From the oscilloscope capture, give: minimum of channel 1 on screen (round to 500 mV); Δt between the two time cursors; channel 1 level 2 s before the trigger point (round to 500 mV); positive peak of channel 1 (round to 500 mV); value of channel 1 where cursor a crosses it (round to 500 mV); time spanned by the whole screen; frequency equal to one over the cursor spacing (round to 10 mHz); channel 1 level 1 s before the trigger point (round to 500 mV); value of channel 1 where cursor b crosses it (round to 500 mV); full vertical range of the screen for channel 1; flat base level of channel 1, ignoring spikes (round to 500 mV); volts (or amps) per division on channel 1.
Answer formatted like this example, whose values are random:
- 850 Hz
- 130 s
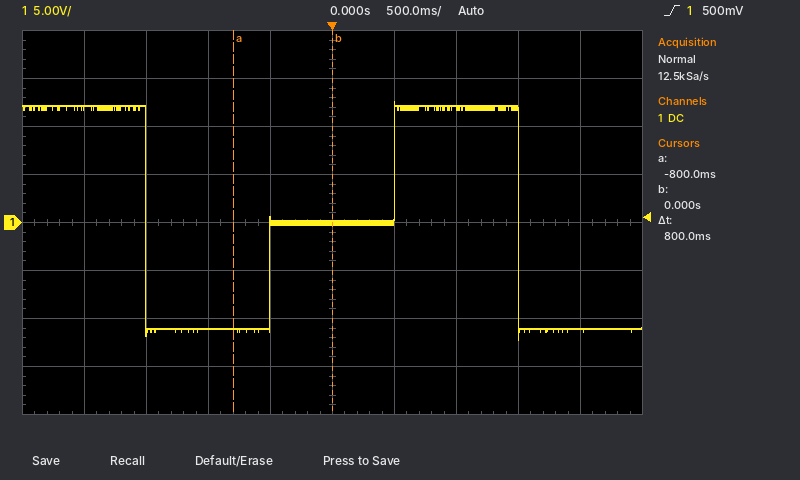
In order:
- -12.0 V
- 800 ms
- 12.0 V
- 12.5 V
- -11.0 V
- 5 s
- 1.25 Hz
- -11.0 V
- 0.0 V
- 40 V
- -11.0 V
- 5 V
